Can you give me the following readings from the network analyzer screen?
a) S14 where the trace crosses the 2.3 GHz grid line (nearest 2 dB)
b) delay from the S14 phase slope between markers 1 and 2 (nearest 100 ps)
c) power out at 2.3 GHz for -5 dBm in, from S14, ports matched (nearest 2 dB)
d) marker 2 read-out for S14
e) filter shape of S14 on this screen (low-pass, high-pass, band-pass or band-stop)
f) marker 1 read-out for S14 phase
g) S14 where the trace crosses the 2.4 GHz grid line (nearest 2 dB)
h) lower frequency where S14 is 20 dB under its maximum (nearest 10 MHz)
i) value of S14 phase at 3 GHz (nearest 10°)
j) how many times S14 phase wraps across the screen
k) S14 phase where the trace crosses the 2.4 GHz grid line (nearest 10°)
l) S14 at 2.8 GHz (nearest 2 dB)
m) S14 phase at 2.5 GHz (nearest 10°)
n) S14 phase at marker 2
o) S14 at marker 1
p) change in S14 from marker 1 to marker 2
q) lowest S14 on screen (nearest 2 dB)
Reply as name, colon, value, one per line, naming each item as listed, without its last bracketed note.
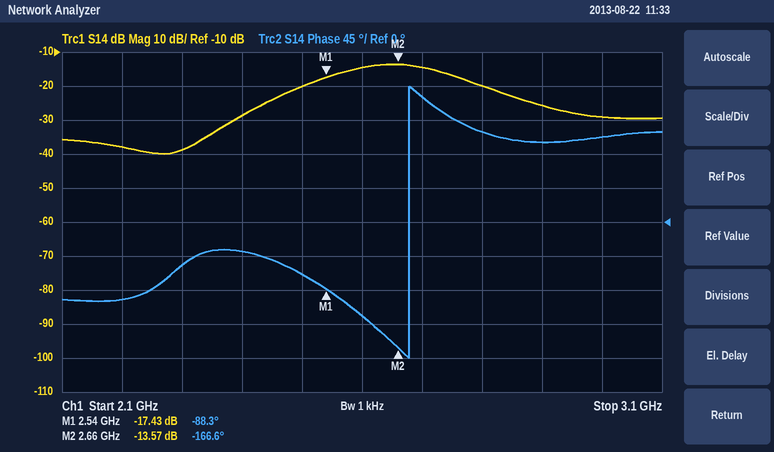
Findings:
S14 where the trace crosses the 2.3 GHz grid line: -38 dB
delay from the S14 phase slope between markers 1 and 2: 1.8 ns
power out at 2.3 GHz for -5 dBm in, from S14, ports matched: -44 dBm
marker 2 read-out for S14: -13.57 dB
filter shape of S14 on this screen: band-pass
marker 1 read-out for S14 phase: -88.3°
S14 where the trace crosses the 2.4 GHz grid line: -28 dB
lower frequency where S14 is 20 dB under its maximum: 2.35 GHz
value of S14 phase at 3 GHz: 110°
how many times S14 phase wraps across the screen: 1
S14 phase where the trace crosses the 2.4 GHz grid line: -40°
S14 at 2.8 GHz: -20 dB
S14 phase at 2.5 GHz: -70°
S14 phase at marker 2: -166.6°
S14 at marker 1: -17.43 dB
change in S14 from marker 1 to marker 2: 3.86 dB
lowest S14 on screen: -40 dB
